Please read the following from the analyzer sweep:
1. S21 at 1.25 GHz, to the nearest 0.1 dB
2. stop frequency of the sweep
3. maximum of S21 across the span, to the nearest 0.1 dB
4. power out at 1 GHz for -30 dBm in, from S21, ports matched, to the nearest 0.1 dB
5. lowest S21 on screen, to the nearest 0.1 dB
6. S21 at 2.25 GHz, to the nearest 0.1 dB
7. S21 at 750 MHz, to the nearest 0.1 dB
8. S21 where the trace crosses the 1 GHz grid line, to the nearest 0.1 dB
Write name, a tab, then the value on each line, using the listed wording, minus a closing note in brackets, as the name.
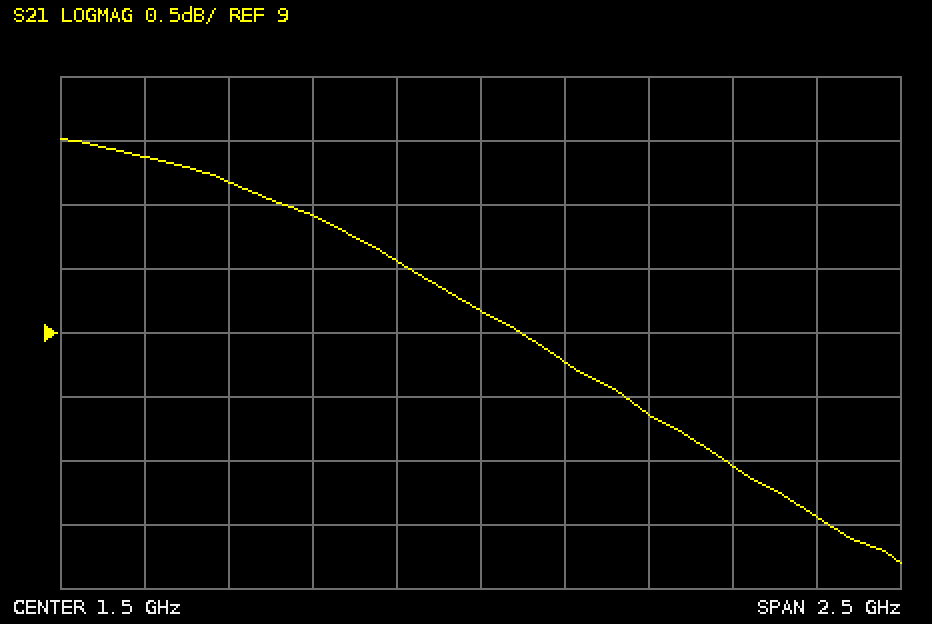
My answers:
S21 at 1.25 GHz, to the nearest 0.1 dB	9.6 dB
stop frequency of the sweep	2.75 GHz
maximum of S21 across the span, to the nearest 0.1 dB	10.5 dB
power out at 1 GHz for -30 dBm in, from S21, ports matched, to the nearest 0.1 dB	-20.1 dBm
lowest S21 on screen, to the nearest 0.1 dB	7.2 dB
S21 at 2.25 GHz, to the nearest 0.1 dB	8.0 dB
S21 at 750 MHz, to the nearest 0.1 dB	10.2 dB
S21 where the trace crosses the 1 GHz grid line, to the nearest 0.1 dB	9.9 dB
